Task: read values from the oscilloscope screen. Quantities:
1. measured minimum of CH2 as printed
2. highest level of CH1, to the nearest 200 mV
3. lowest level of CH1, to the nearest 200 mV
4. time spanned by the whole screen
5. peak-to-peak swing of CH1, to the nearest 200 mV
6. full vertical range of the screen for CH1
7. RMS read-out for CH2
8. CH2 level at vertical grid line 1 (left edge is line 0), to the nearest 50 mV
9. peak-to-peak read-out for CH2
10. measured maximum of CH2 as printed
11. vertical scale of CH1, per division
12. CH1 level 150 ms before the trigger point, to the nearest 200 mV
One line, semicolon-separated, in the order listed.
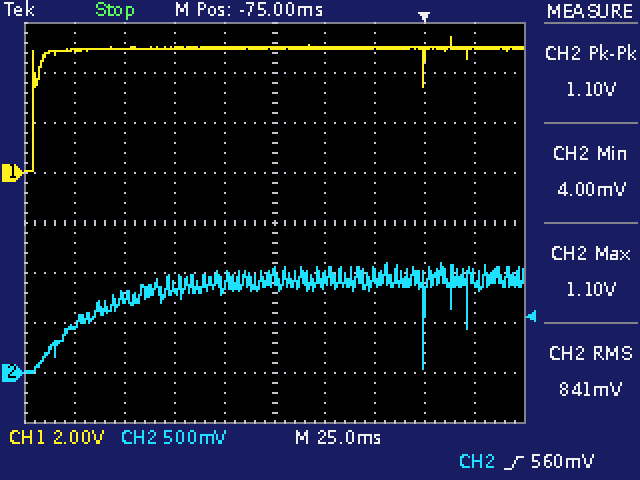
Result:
4.00 mV; 5.4 V; 0.0 V; 250 ms; 5.4 V; 16 V; 841 mV; 500 mV; 1.10 V; 1.10 V; 2 V; 5.0 V
